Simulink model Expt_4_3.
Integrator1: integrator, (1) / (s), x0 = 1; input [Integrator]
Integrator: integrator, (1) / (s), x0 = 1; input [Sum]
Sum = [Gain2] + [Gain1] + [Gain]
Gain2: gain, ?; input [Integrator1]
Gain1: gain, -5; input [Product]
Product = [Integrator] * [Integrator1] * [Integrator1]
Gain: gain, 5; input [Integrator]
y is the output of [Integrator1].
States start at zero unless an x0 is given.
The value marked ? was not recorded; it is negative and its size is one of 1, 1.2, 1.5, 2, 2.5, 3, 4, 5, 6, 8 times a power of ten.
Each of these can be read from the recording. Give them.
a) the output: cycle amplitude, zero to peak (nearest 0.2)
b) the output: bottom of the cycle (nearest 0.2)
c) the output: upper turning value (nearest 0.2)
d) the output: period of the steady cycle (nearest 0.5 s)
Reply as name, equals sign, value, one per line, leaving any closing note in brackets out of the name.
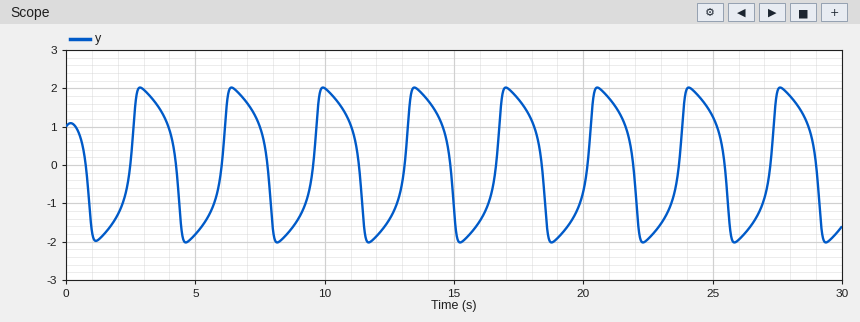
the output: cycle amplitude, zero to peak = 2.0
the output: bottom of the cycle = -2.0
the output: upper turning value = 2.0
the output: period of the steady cycle = 3.5 s
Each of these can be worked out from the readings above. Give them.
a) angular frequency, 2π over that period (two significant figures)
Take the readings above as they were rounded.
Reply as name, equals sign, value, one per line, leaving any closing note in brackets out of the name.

angular frequency, 2π over that period = 1.8 rad/s
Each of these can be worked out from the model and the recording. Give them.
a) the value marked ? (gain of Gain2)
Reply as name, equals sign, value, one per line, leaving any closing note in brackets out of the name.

the value marked ? = -5
